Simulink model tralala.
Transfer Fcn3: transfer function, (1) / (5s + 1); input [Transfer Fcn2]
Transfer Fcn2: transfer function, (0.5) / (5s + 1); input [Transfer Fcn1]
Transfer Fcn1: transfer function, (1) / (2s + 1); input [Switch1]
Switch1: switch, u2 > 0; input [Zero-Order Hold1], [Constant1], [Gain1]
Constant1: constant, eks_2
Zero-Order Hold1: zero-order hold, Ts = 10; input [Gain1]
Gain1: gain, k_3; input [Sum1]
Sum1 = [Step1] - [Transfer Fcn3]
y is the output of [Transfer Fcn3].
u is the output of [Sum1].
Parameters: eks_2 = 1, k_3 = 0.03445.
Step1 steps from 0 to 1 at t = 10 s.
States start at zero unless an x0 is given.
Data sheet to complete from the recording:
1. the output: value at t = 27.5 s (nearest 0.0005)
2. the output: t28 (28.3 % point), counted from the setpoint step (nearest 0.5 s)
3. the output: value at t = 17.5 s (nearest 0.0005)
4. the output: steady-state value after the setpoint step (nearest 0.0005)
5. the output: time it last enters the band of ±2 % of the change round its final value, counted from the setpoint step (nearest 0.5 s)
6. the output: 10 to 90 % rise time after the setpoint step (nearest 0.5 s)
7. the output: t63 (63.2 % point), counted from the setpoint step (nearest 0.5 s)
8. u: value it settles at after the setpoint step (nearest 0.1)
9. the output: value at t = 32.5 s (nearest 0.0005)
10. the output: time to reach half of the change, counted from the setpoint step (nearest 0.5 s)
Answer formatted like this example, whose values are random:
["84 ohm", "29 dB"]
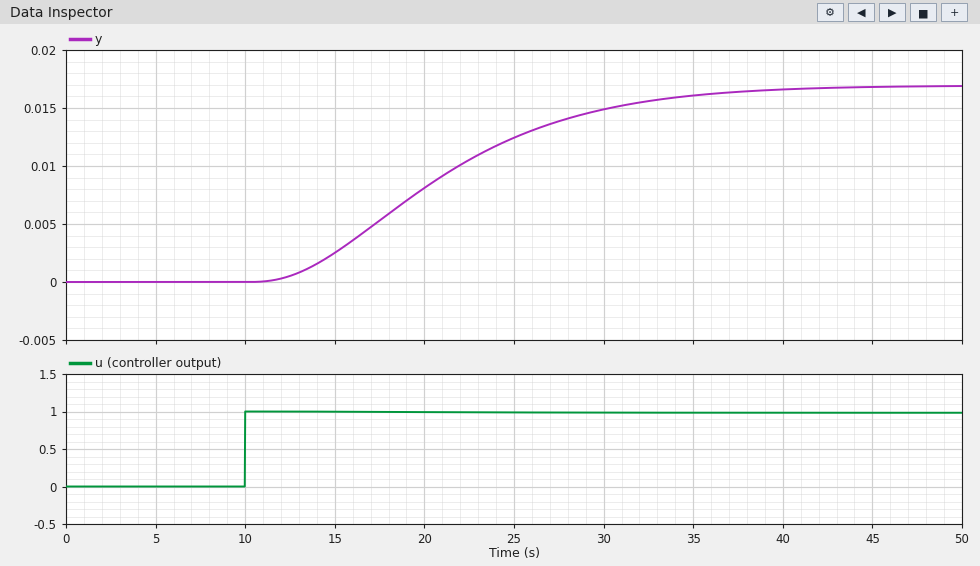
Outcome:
["0.0140", "7.0 s", "0.0055", "0.0170", "30.0 s", "17.0 s", "12.5 s", "1.0", "0.0155", "10.5 s"]
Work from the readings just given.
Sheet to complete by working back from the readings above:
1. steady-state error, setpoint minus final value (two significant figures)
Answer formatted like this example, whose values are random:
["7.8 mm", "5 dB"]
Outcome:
["0.98"]
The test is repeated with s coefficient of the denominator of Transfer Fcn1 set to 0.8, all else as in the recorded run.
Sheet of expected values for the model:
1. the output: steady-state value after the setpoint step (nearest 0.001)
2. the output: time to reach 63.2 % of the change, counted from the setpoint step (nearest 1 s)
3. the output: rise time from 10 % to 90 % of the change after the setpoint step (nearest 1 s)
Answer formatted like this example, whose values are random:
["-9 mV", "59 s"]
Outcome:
["0.017", "11 s", "16 s"]
